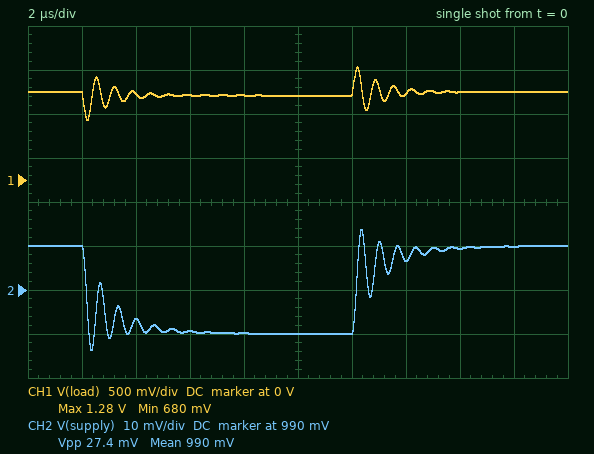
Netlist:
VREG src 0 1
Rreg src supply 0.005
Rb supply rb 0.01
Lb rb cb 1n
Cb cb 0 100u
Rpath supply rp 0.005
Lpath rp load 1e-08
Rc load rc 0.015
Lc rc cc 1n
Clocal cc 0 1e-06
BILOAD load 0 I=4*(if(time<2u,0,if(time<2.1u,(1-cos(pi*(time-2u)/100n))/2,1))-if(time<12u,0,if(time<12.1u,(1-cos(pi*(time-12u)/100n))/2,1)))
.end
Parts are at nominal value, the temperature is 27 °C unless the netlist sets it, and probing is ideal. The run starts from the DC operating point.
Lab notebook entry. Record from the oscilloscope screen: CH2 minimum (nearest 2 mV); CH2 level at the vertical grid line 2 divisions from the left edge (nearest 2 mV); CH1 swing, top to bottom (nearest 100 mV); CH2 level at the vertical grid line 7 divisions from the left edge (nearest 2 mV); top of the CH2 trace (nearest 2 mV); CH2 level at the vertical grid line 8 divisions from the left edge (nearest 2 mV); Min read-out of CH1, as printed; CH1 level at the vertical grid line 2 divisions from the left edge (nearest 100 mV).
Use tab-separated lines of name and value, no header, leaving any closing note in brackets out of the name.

CH2 minimum	976 mV
CH2 level at the vertical grid line 2 divisions from the left edge	984 mV
CH1 swing, top to bottom	600 mV
CH2 level at the vertical grid line 7 divisions from the left edge	996 mV
top of the CH2 trace	1.004 V
CH2 level at the vertical grid line 8 divisions from the left edge	1.000 V
Min read-out of CH1, as printed	680 mV
CH1 level at the vertical grid line 2 divisions from the left edge	1.0 V
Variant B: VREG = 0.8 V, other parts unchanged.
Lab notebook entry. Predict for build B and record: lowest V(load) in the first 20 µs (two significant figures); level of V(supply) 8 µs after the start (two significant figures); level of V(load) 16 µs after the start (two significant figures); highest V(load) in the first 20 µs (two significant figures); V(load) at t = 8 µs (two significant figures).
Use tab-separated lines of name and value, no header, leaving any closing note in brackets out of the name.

lowest V(load) in the first 20 µs	480 mV
level of V(supply) 8 µs after the start	780 mV
level of V(load) 16 µs after the start	800 mV
highest V(load) in the first 20 µs	1.1 V
V(load) at t = 8 µs	760 mV
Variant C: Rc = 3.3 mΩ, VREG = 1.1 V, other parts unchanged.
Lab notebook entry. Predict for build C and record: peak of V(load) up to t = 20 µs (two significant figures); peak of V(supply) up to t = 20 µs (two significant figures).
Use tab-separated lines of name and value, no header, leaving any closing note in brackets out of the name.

peak of V(load) up to t = 20 µs	1.4 V
peak of V(supply) up to t = 20 µs	1.1 V
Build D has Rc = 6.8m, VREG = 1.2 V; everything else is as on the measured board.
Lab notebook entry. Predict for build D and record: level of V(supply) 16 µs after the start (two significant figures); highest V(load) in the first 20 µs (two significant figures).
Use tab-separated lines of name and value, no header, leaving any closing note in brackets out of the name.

level of V(supply) 16 µs after the start	1.2 V
highest V(load) in the first 20 µs	1.5 V
